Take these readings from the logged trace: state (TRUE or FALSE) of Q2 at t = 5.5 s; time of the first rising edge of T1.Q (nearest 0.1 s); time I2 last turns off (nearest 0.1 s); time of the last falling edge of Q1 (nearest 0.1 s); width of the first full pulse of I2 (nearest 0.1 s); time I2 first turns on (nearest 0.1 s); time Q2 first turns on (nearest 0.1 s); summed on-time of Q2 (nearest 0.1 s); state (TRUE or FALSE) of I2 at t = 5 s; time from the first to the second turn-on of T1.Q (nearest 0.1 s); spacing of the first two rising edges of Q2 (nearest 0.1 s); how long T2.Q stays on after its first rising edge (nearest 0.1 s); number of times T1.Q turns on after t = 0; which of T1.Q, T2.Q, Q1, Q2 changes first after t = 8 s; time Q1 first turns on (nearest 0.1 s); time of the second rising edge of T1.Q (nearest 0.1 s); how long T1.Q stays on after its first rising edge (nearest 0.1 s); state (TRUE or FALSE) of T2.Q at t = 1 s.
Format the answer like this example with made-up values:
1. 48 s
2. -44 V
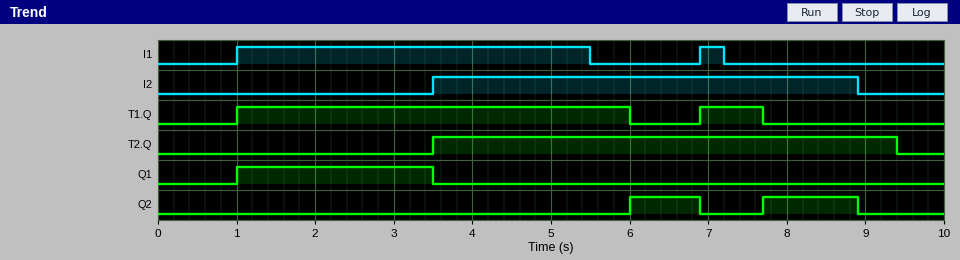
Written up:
1. FALSE
2. 1.0 s
3. 8.9 s
4. 3.5 s
5. 5.4 s
6. 3.5 s
7. 6.0 s
8. 2.1 s
9. TRUE
10. 5.9 s
11. 1.7 s
12. 5.9 s
13. 2
14. Q2
15. 1.0 s
16. 6.9 s
17. 5.0 s
18. FALSE
